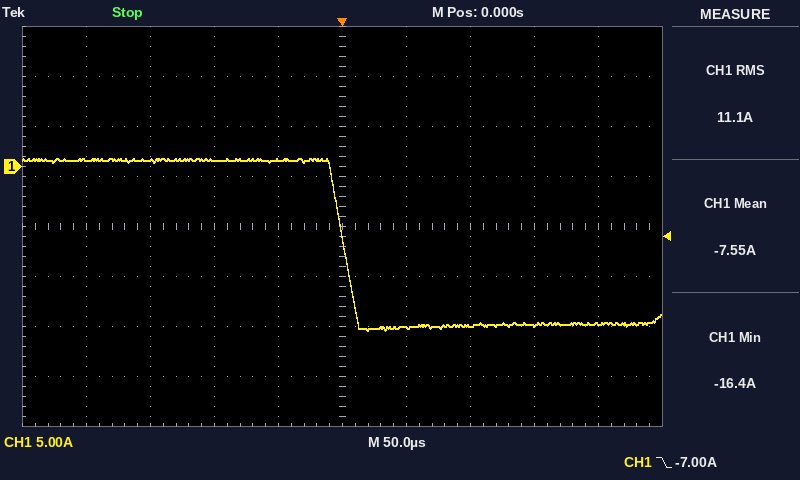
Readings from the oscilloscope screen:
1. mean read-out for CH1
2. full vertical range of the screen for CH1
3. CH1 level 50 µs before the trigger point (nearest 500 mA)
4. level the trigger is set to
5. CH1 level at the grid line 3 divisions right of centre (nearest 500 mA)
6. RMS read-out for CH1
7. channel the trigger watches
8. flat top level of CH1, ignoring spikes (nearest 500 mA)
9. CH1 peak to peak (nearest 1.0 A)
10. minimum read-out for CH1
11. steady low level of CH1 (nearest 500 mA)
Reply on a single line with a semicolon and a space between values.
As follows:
-7.55 A; 40 A; 500 mA; -7.00 A; -16.0 A; 11.1 A; CH1; 500 mA; 17.0 A; -16.4 A; -16.0 A
